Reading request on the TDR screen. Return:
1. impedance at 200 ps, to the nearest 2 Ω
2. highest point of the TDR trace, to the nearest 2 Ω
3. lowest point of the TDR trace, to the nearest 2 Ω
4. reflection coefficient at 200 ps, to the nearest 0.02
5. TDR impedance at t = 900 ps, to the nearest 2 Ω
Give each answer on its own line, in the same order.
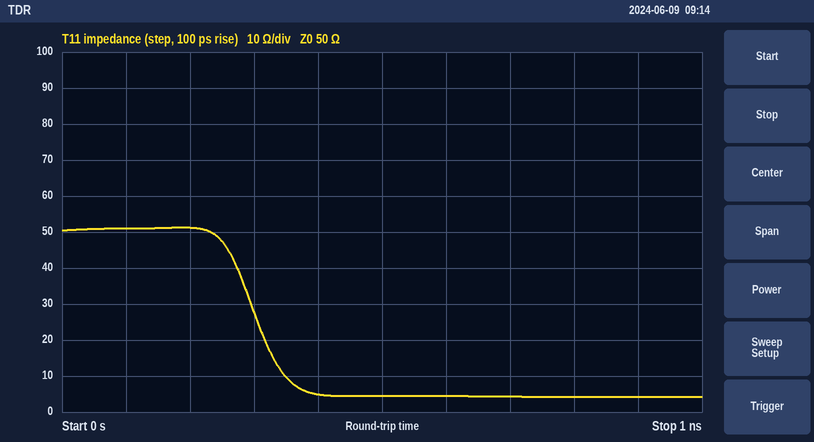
52 Ω
52 Ω
4 Ω
+0.02
4 Ω
